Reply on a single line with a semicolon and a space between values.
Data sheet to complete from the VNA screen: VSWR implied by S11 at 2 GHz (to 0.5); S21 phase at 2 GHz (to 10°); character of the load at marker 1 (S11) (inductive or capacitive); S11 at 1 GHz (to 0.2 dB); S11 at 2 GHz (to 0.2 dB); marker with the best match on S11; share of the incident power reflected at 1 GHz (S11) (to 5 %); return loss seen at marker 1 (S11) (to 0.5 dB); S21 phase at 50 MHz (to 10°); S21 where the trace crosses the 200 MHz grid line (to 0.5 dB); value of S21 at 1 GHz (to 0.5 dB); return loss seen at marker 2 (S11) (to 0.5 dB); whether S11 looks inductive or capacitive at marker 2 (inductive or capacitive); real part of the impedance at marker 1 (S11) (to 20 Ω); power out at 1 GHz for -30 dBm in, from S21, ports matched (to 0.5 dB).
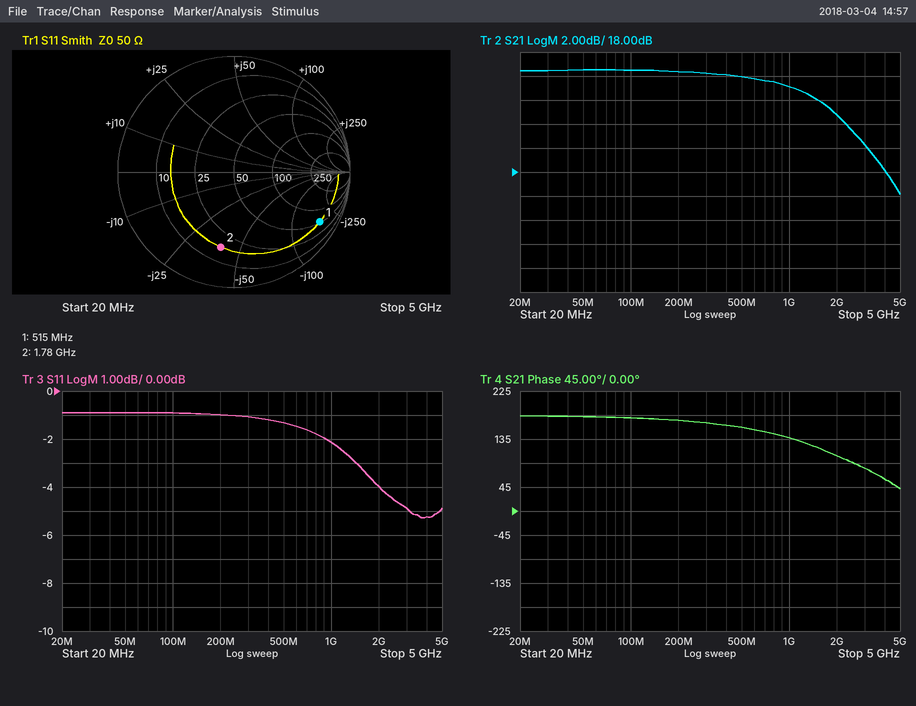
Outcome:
4.5; 100°; capacitive; -2.2 dB; -4.0 dB; marker 2; 60 %; 1.5 dB; 180°; 26.5 dB; 25.0 dB; 3.5 dB; capacitive; 60 Ω; -5.0 dBm
